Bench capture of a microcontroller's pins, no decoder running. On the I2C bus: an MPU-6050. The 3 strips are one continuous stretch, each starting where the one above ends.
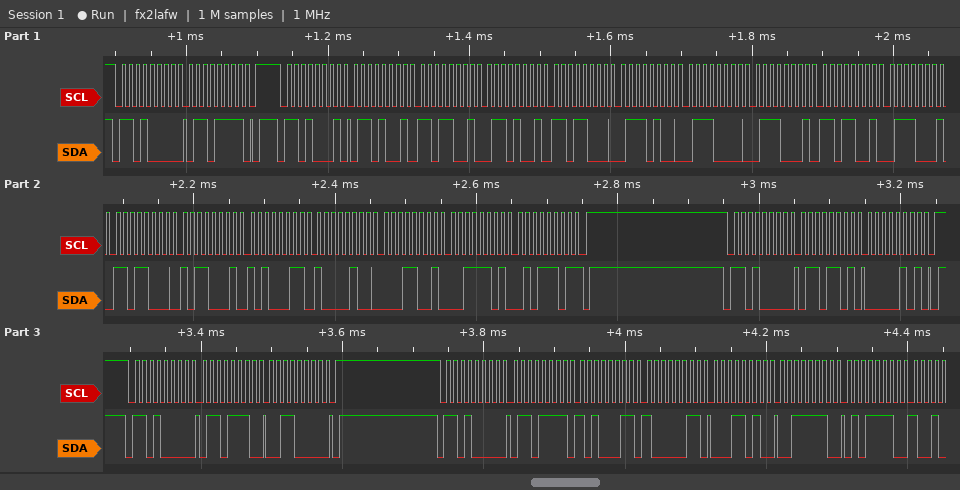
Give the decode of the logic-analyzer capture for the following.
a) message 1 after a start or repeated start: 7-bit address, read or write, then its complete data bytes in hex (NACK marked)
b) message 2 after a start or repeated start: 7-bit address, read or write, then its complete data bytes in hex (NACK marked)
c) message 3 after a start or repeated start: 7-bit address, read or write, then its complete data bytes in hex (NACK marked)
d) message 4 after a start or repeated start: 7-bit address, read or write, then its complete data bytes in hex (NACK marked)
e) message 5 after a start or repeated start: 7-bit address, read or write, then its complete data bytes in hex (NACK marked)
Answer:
0x68 write: 6F
0x68 read: 69 D9 69 D8 74 70 71 D9 71 D8 B1 A3 84 19 3D 5D NACK
0x68 write: 6D 05
0x68 write: 6E 30
0x68 write: 6F A3 83 1A 3E 5E
